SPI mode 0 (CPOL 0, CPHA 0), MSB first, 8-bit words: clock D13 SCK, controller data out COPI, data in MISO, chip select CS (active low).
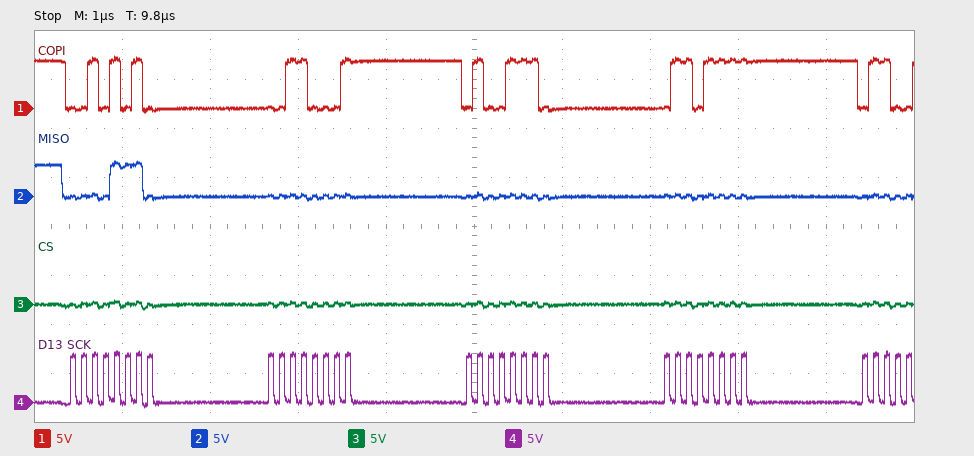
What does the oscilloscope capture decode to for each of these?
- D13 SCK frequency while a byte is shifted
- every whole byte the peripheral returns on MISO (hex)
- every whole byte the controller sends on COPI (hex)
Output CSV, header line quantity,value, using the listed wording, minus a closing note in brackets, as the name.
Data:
quantity,value
D13 SCK frequency while a byte is shifted,8 MHz
every whole byte the peripheral returns on MISO,0E 00 00 00
every whole byte the controller sends on COPI,2A 31 4E 6F
